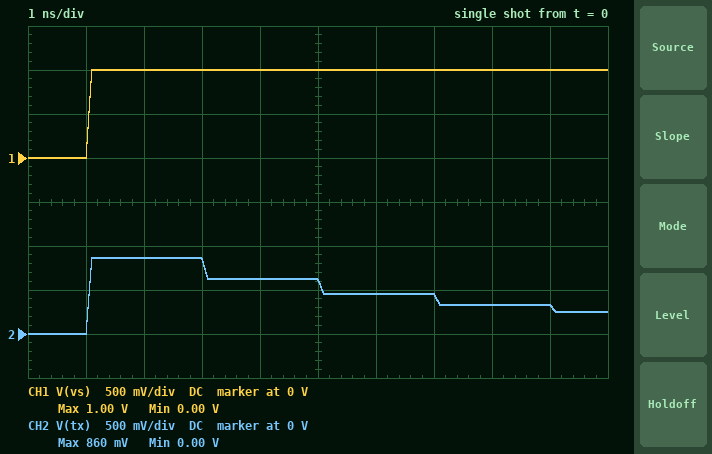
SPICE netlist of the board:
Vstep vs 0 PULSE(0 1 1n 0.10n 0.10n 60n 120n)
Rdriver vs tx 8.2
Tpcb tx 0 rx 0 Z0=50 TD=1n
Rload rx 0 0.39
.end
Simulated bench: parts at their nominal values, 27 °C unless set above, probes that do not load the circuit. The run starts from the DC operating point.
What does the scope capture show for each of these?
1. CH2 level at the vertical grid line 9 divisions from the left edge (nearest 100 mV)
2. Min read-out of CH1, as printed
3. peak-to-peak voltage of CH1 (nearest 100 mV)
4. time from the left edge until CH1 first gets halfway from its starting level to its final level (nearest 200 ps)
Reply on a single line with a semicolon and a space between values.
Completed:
300 mV; 0.00 V; 1.0 V; 1.0 ns
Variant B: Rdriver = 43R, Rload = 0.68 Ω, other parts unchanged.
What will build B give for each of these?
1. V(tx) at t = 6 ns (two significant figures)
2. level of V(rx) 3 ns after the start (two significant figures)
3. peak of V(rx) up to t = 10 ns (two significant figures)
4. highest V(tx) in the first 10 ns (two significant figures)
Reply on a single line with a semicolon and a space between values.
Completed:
18 mV; 14 mV; 16 mV; 540 mV
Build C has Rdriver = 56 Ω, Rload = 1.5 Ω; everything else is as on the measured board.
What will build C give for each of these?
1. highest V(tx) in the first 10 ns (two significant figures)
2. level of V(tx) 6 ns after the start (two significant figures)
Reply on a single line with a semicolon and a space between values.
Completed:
470 mV; 27 mV
